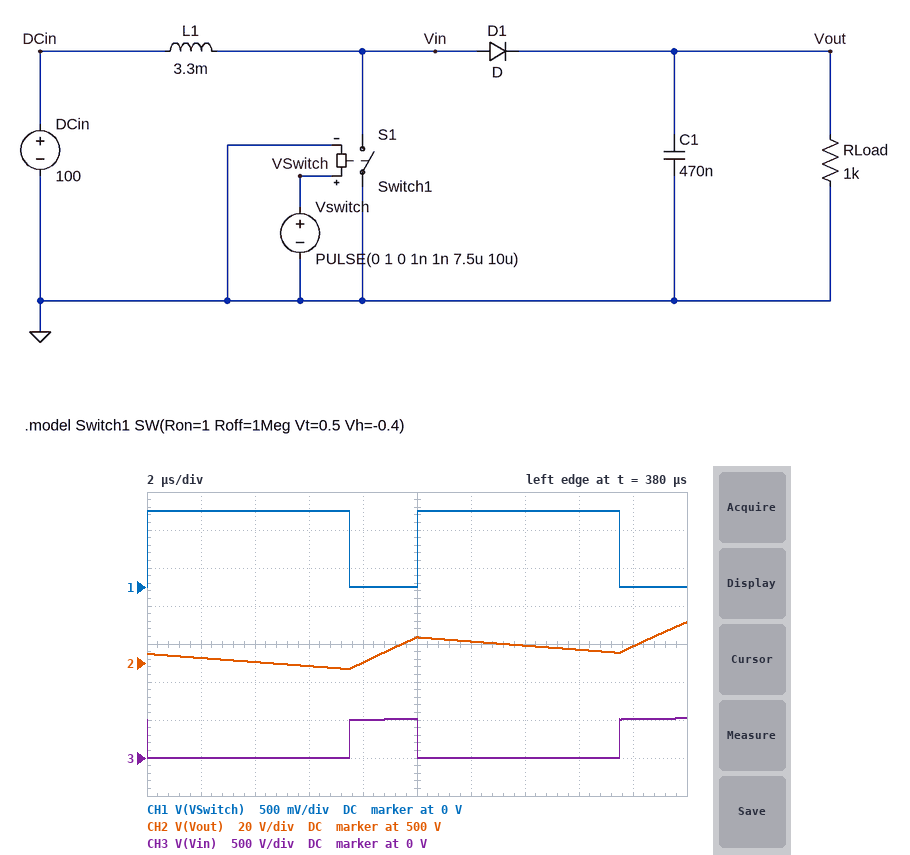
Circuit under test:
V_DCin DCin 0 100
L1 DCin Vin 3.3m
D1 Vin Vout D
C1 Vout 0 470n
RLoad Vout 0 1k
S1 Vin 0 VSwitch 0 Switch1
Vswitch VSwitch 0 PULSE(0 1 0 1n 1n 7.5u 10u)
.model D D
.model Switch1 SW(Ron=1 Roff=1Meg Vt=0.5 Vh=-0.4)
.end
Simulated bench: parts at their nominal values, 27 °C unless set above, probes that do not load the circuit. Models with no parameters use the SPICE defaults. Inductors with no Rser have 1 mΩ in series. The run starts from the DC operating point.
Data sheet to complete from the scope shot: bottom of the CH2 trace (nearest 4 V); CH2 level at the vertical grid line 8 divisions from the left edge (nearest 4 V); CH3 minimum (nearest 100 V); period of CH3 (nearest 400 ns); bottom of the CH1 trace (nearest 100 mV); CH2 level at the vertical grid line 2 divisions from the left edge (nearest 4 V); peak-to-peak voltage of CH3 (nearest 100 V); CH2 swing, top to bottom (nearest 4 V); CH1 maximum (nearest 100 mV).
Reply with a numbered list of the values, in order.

1. 496 V
2. 508 V
3. 0 V
4. 10.0 µs
5. 0 V
6. 500 V
7. 500 V
8. 24 V
9. 1.0 V
